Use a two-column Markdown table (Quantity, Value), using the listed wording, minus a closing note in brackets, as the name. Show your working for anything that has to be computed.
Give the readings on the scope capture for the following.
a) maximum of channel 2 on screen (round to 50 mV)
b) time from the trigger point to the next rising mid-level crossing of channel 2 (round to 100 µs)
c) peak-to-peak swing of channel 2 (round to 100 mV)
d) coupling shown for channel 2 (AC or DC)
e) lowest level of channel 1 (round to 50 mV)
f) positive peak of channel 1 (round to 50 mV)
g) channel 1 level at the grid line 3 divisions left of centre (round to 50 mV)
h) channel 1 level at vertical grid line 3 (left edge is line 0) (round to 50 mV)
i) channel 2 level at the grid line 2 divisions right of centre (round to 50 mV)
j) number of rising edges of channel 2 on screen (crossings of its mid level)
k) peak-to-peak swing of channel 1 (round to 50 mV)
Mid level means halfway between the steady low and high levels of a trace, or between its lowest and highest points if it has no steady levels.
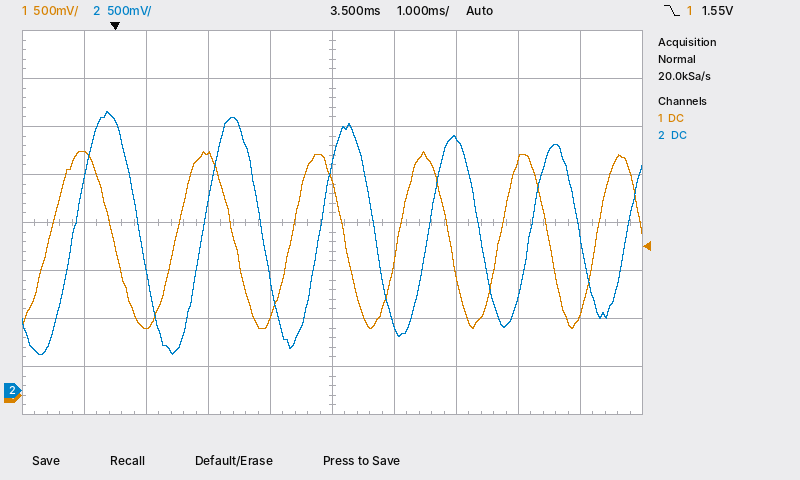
| Quantity | Value |
|---|---|
| maximum of channel 2 on screen | 2.90 V |
| time from the trigger point to the next rising mid-level crossing of channel 2 | 1.4 ms |
| peak-to-peak swing of channel 2 | 2.50 V |
| coupling shown for channel 2 | DC |
| lowest level of channel 1 | 700 mV |
| positive peak of channel 1 | 2.55 V |
| channel 1 level at the grid line 3 divisions left of centre | 700 mV |
| channel 1 level at vertical grid line 3 (left edge is line 0) | 2.50 V |
| channel 2 level at the grid line 2 divisions right of centre | 2.60 V |
| number of rising edges of channel 2 on screen | 6 |
| peak-to-peak swing of channel 1 | 2.55 V − (700 mV) = 1.85 V |
